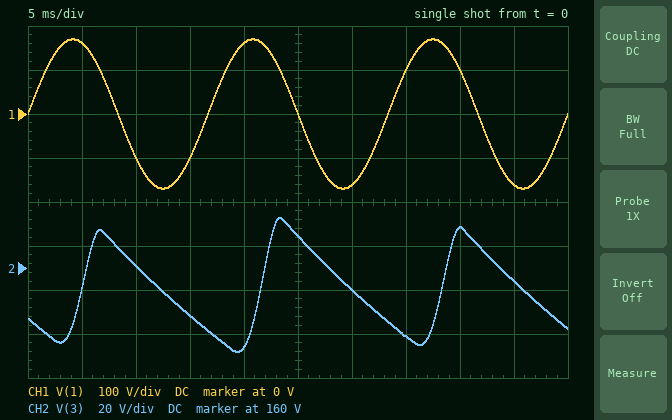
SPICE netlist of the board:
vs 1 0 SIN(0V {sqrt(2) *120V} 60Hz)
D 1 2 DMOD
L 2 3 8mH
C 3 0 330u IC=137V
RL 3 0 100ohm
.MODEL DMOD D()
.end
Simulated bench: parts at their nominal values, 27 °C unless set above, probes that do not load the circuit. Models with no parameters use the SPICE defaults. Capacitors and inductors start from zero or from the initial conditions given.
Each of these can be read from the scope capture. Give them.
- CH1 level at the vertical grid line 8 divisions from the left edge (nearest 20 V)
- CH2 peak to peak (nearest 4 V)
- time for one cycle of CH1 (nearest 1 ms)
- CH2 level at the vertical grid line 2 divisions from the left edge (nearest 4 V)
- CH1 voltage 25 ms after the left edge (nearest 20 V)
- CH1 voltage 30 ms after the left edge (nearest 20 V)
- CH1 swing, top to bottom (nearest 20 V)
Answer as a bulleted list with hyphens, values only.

- 100 V
- 60 V
- 17 ms
- 160 V
- 0 V
- -160 V
- 340 V
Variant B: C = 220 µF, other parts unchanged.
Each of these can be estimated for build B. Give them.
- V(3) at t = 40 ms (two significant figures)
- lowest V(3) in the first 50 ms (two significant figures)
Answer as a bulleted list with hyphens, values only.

- 200 V
- 110 V
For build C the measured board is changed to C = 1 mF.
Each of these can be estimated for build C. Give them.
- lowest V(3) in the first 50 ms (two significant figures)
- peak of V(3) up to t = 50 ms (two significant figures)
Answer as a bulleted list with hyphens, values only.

- 130 V
- 150 V
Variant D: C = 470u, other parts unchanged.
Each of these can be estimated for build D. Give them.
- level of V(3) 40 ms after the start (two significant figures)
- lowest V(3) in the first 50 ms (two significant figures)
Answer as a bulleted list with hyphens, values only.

- 170 V
- 130 V
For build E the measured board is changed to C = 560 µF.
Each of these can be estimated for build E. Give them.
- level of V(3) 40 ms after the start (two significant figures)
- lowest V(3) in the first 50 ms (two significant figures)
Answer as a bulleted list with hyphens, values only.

- 160 V
- 130 V
